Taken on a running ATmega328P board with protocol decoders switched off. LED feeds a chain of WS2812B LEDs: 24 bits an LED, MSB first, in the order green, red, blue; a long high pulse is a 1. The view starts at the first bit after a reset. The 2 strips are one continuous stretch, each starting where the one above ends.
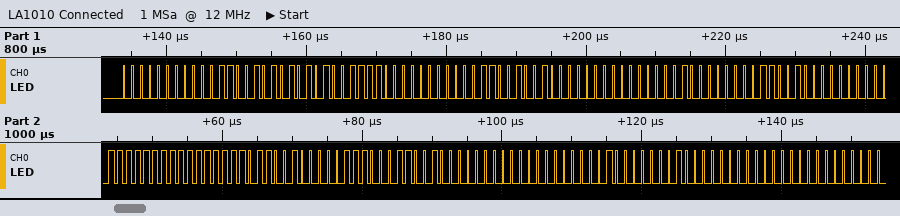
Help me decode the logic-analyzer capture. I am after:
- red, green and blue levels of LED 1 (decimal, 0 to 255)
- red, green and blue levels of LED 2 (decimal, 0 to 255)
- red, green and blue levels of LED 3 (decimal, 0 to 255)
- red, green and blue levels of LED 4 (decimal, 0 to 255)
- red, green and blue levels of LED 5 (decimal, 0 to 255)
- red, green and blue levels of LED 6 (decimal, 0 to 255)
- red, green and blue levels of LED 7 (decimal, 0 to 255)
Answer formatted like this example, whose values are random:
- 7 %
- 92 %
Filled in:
- 25, 0, 85
- 0, 60, 100
- 0, 128, 128
- 0, 100, 255
- 100, 255, 28
- 0, 100, 0
- 64, 64, 0
